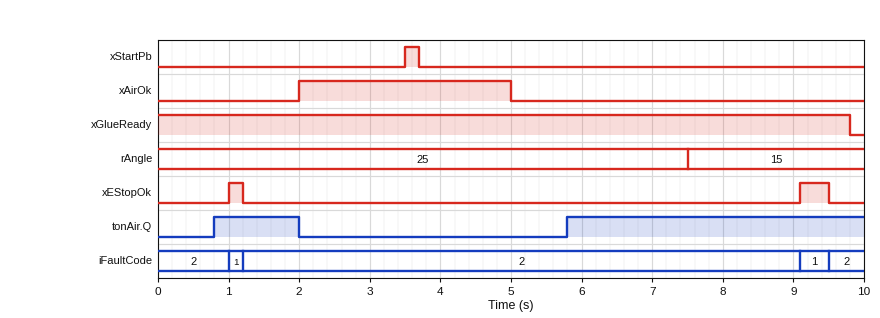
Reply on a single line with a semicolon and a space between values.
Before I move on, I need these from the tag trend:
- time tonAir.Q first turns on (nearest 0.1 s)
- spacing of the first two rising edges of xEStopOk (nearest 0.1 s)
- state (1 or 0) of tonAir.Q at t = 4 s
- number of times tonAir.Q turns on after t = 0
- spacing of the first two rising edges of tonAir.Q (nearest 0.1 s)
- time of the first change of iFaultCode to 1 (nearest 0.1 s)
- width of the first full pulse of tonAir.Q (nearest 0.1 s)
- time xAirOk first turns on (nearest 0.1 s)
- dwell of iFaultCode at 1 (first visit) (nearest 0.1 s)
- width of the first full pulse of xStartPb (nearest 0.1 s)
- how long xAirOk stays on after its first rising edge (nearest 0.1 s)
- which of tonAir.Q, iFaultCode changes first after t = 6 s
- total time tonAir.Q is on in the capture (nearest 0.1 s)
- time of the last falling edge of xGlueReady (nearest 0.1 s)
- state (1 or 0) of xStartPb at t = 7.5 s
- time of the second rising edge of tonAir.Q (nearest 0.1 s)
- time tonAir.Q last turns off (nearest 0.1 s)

0.8 s; 8.1 s; 0; 2; 5.0 s; 1.0 s; 1.2 s; 2.0 s; 0.2 s; 0.2 s; 3.0 s; iFaultCode; 5.4 s; 9.8 s; 0; 5.8 s; 2.0 s
